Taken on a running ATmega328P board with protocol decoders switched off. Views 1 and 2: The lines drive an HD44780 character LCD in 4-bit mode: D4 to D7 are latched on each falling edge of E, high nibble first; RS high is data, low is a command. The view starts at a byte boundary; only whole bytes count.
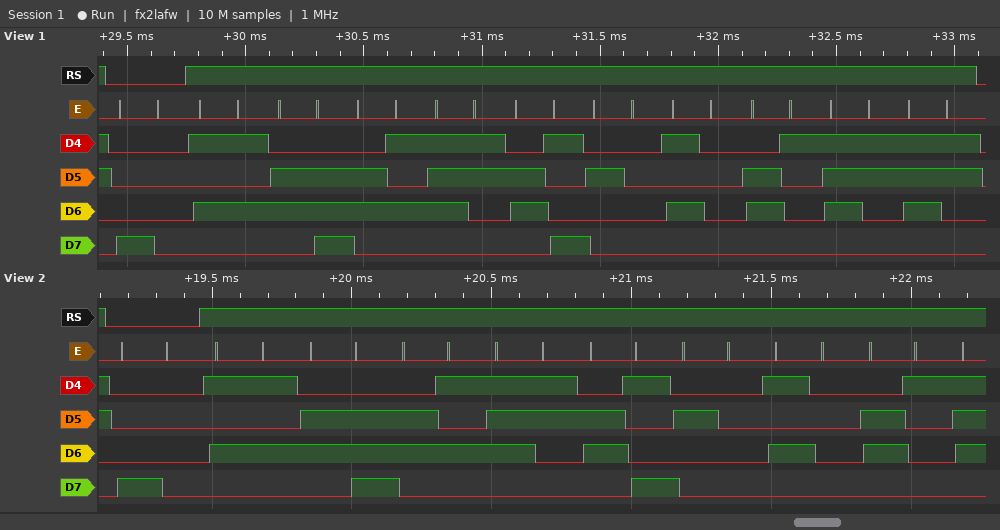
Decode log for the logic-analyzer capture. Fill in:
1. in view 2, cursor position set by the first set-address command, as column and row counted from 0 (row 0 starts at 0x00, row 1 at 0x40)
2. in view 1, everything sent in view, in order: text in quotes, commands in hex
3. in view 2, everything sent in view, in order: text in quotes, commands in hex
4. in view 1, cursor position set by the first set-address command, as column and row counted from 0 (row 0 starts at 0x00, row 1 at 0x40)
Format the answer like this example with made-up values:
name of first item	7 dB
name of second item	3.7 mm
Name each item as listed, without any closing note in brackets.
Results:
in view 2, cursor position set by the first set-address command, as column and row counted from 0	column 0, row 0
in view 1, everything sent in view, in order: text in quotes, commands in hex	0x80 "Unesi Pass"
in view 2, everything sent in view, in order: text in quotes, commands in hex	0x80 "Unesi Pa"
in view 1, cursor position set by the first set-address command, as column and row counted from 0	column 0, row 0
